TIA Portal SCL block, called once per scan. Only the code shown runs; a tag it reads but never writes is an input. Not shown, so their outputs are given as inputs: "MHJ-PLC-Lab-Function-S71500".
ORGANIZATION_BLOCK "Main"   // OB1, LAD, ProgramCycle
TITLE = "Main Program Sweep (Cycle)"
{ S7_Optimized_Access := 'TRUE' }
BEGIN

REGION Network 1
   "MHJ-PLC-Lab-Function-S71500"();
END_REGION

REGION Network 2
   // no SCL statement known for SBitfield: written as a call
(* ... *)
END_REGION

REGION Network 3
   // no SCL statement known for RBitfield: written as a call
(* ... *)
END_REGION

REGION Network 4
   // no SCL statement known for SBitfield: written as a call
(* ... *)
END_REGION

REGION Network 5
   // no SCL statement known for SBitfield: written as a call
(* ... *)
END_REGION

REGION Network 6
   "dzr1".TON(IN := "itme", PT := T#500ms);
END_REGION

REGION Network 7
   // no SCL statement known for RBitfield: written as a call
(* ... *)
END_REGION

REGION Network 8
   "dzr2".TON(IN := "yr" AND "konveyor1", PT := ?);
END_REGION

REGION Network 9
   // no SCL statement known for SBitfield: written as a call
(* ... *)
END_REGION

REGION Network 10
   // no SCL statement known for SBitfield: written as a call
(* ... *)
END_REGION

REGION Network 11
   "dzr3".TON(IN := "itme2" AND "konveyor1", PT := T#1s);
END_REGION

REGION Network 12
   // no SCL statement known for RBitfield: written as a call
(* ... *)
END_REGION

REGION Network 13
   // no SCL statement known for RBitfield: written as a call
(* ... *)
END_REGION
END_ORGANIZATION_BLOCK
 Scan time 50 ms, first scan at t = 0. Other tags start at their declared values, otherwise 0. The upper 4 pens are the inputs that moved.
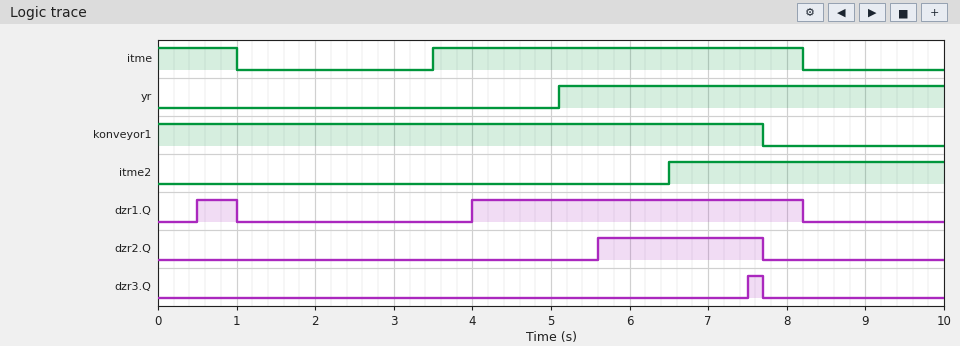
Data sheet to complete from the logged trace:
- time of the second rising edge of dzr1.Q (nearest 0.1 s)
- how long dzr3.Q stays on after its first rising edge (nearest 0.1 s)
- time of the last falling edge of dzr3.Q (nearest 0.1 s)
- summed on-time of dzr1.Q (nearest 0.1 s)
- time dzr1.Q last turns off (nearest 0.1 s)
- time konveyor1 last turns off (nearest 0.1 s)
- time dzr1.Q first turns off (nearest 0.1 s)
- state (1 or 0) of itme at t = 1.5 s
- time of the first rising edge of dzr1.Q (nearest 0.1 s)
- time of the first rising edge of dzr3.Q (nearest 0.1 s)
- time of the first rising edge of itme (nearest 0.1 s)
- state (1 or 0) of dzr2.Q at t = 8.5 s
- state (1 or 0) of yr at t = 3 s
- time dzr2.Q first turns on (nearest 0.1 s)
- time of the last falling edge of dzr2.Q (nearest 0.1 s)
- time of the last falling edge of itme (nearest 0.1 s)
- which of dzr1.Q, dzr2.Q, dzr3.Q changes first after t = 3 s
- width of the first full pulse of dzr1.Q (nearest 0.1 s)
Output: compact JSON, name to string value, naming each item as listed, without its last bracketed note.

{"time of the second rising edge of dzr1.Q": "4.0 s", "how long dzr3.Q stays on after its first rising edge": "0.2 s", "time of the last falling edge of dzr3.Q": "7.7 s", "summed on-time of dzr1.Q": "4.7 s", "time dzr1.Q last turns off": "8.2 s", "time konveyor1 last turns off": "7.7 s", "time dzr1.Q first turns off": "1.0 s", "state (1 or 0) of itme at t = 1.5 s": "0", "time of the first rising edge of dzr1.Q": "0.5 s", "time of the first rising edge of dzr3.Q": "7.5 s", "time of the first rising edge of itme": "3.5 s", "state (1 or 0) of dzr2.Q at t = 8.5 s": "0", "state (1 or 0) of yr at t = 3 s": "0", "time dzr2.Q first turns on": "5.6 s", "time of the last falling edge of dzr2.Q": "7.7 s", "time of the last falling edge of itme": "8.2 s", "which of dzr1.Q, dzr2.Q, dzr3.Q changes first after t = 3 s": "dzr1.Q", "width of the first full pulse of dzr1.Q": "0.5 s"}
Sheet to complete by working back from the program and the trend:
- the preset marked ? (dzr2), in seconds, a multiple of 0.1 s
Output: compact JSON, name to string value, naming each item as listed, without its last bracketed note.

{"the preset marked ? (dzr2), in seconds, a multiple of 0.1 s": "0.5 s"}
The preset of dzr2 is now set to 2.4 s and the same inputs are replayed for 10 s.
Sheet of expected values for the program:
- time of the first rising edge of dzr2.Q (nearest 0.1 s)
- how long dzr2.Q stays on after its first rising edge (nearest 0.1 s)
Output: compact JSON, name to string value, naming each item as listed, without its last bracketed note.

{"time of the first rising edge of dzr2.Q": "7.5 s", "how long dzr2.Q stays on after its first rising edge": "0.2 s"}
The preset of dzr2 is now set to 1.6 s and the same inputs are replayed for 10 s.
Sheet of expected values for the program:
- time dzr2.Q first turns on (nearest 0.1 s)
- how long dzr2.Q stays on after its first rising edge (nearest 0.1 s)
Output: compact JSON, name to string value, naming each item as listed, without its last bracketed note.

{"time dzr2.Q first turns on": "6.7 s", "how long dzr2.Q stays on after its first rising edge": "1.0 s"}
